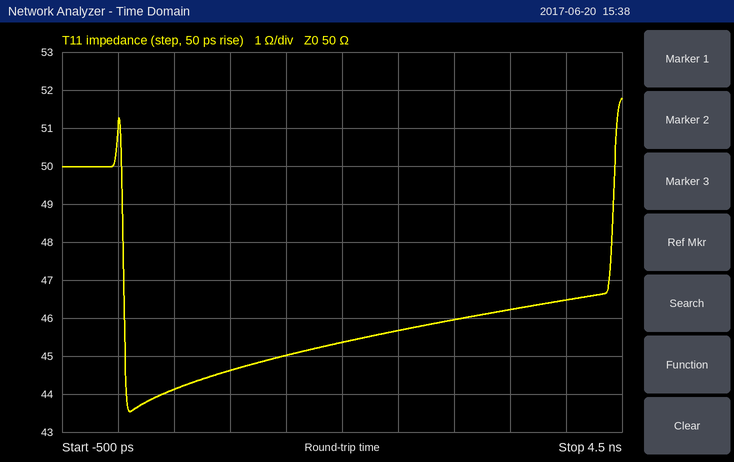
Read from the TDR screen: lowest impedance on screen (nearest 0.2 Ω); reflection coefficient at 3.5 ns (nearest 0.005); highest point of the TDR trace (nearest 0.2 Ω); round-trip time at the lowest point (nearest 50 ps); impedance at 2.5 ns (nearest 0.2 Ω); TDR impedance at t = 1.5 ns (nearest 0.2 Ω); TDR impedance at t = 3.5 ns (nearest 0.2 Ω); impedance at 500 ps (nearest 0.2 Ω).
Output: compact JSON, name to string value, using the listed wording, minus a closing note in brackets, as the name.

{"lowest impedance on screen": "43.6 Ω", "reflection coefficient at 3.5 ns": "-0.040", "highest point of the TDR trace": "51.8 Ω", "round-trip time at the lowest point": "100 ps", "impedance at 2.5 ns": "45.6 Ω", "TDR impedance at t = 1.5 ns": "45.0 Ω", "TDR impedance at t = 3.5 ns": "46.2 Ω", "impedance at 500 ps": "44.2 Ω"}
